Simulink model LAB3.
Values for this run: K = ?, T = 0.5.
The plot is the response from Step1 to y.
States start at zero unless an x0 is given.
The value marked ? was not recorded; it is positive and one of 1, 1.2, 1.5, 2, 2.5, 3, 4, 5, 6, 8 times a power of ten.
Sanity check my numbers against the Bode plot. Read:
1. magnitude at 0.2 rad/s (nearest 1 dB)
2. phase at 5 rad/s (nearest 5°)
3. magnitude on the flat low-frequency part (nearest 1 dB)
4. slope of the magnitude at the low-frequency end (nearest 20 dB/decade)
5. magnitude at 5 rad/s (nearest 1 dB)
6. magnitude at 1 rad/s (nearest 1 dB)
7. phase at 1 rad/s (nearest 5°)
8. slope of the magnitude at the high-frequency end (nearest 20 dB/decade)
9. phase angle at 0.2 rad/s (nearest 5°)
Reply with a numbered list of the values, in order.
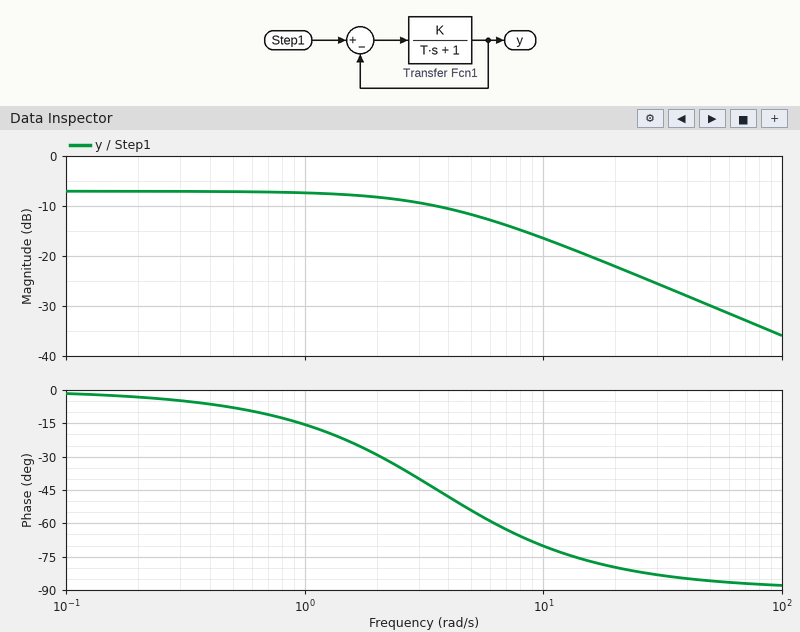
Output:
1. -7 dB
2. -55°
3. -7 dB
4. 0 dB/decade
5. -12 dB
6. -7 dB
7. -15°
8. -20 dB/decade
9. -5°
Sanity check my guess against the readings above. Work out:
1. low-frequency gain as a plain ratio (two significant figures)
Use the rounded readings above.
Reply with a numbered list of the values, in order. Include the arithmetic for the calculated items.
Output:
1. 10^(-7 / 20) = 0.45
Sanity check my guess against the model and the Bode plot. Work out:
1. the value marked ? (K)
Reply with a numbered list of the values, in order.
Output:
1. 0.8
